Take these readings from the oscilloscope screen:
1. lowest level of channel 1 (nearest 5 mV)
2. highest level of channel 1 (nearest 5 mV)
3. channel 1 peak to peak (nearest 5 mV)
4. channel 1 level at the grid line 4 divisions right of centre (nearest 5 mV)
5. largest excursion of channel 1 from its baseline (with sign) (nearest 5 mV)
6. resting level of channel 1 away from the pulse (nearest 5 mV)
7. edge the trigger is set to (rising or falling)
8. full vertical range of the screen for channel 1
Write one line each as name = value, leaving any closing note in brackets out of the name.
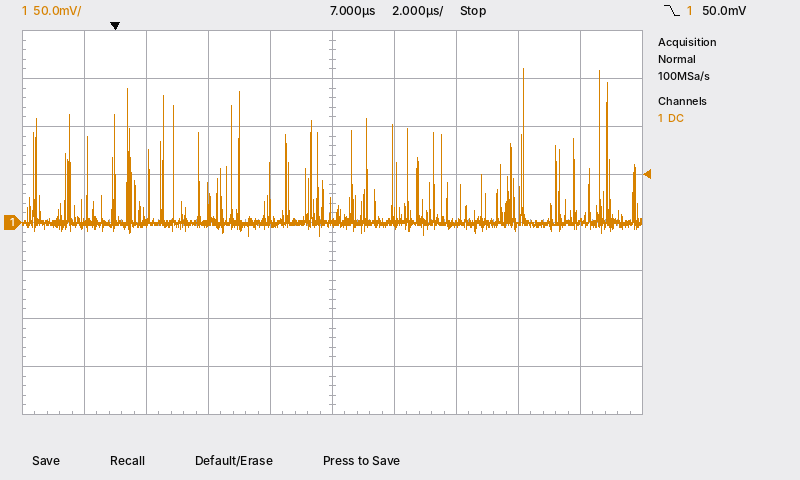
lowest level of channel 1 = -15 mV
highest level of channel 1 = 160 mV
channel 1 peak to peak = 175 mV
channel 1 level at the grid line 4 divisions right of centre = 0 mV
largest excursion of channel 1 from its baseline (with sign) = +160 mV
resting level of channel 1 away from the pulse = 0 mV
edge the trigger is set to = falling
full vertical range of the screen for channel 1 = 400 mV
